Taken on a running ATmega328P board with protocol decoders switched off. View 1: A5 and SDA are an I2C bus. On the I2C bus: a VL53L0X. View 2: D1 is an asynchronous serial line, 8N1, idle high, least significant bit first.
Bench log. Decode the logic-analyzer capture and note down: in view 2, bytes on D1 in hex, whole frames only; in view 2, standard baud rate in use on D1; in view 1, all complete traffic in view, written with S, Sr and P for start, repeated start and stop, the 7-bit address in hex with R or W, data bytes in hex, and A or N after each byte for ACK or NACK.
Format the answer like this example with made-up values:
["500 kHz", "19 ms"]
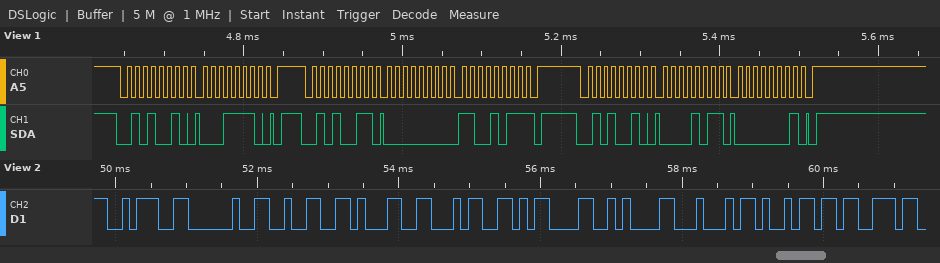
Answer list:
["3A 20 32 31 34 0D 0A 44 69 73", "9600 baud", "S 29W A 1E A P S 29R A 00 A CB N P S 29W A 0B A 01 A P"]
